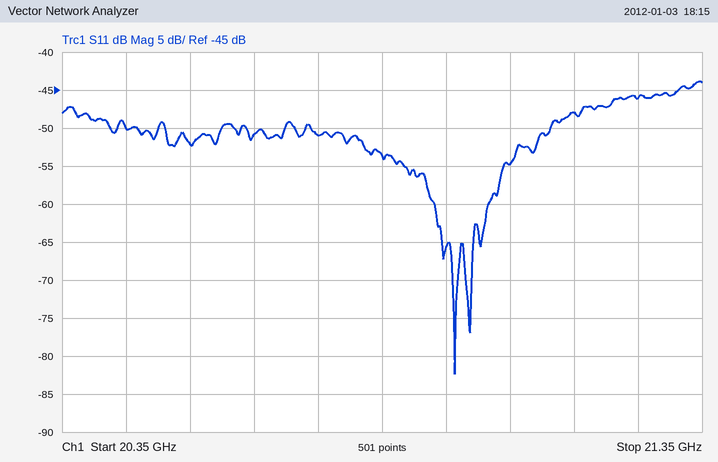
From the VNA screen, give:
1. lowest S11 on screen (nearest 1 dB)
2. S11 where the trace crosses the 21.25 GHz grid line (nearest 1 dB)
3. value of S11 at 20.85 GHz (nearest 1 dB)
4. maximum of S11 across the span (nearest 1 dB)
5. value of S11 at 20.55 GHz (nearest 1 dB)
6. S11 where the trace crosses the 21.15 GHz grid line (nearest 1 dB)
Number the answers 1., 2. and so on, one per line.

1. -82 dB
2. -46 dB
3. -54 dB
4. -44 dB
5. -52 dB
6. -48 dB
